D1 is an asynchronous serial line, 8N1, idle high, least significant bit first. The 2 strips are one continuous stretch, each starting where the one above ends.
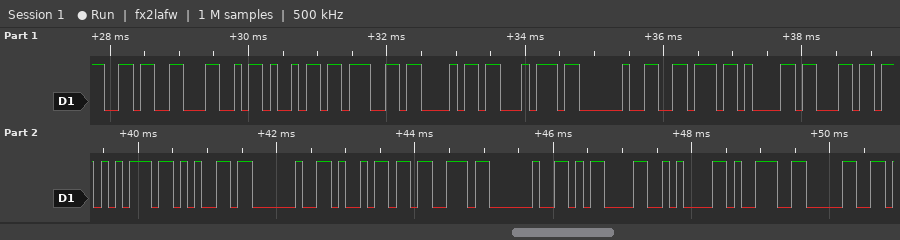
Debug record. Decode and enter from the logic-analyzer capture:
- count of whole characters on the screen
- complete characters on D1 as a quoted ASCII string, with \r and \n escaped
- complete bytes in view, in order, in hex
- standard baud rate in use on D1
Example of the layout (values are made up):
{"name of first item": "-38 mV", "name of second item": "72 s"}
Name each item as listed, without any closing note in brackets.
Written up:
{"count of whole characters on the screen": "20", "complete characters on D1 as a quoted ASCII string, with \\r and \\n escaped": "\"6Light value is \\r\\n90\"", "complete bytes in view, in order, in hex": "36 4C 69 67 68 74 20 76 61 6C 75 65 20 69 73 20 0D 0A 39 30", "standard baud rate in use on D1": "9600 baud"}
